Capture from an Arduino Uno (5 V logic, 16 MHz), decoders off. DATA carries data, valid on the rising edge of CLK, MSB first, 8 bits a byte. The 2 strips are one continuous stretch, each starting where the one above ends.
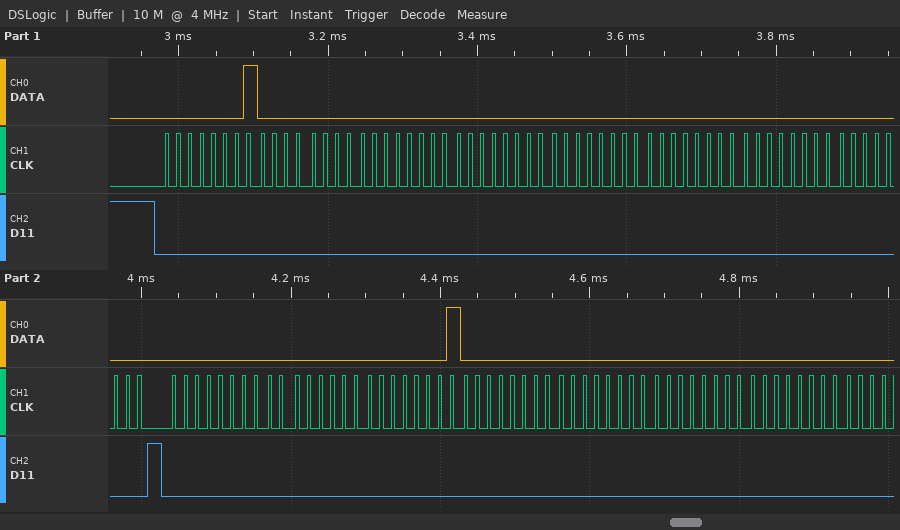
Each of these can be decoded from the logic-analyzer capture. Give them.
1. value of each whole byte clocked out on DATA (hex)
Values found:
0x01 0x00 0x00 0x00 0x00 0x00 0x00 0x00 0x00 0x00 0x01 0x00 0x00 0x00 0x00
